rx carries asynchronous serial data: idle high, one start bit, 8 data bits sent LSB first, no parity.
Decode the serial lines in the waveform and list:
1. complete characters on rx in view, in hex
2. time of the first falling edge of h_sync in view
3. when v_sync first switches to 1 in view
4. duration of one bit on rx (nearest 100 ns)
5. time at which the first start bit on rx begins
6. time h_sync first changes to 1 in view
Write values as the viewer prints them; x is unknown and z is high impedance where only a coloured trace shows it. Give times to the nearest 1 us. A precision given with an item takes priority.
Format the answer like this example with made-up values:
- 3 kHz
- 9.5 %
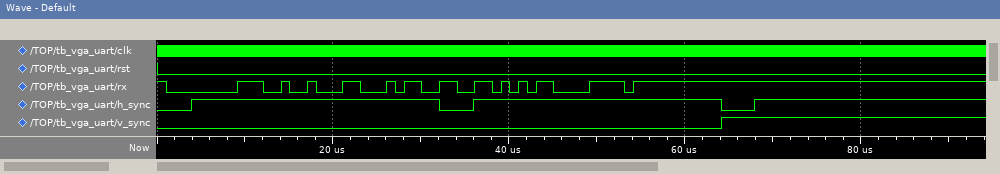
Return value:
- 80, 12, 34, 56, 78
- 32 us
- 64 us
- 1000 ns
- 1 us
- 4 us
